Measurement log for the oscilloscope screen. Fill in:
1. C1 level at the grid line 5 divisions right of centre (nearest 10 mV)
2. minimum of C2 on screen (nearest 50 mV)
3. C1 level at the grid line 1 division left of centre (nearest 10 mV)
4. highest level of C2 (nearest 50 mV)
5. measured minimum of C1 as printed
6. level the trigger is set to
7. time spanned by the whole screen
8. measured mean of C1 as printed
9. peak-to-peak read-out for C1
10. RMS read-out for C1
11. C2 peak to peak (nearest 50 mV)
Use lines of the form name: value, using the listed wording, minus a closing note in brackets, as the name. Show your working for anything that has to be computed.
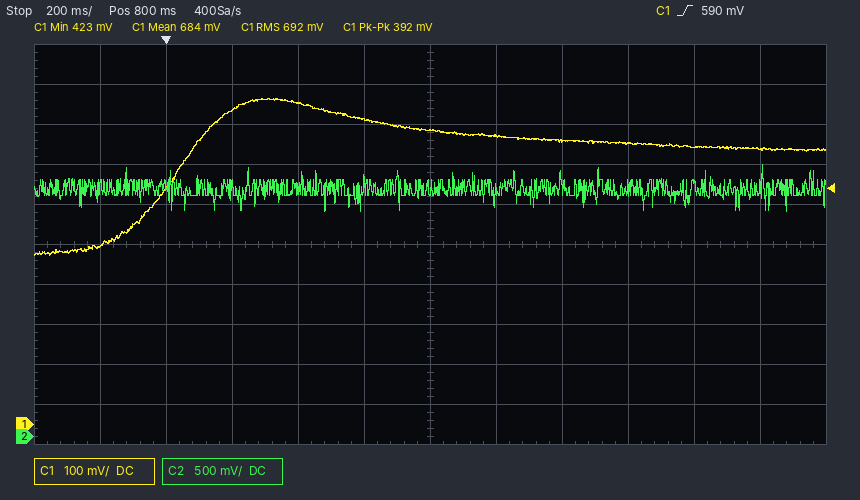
C1 level at the grid line 5 divisions right of centre: 690 mV
minimum of C2 on screen: 2.80 V
C1 level at the grid line 1 division left of centre: 760 mV
highest level of C2: 3.40 V
measured minimum of C1 as printed: 423 mV
level the trigger is set to: 590 mV
time spanned by the whole screen: 2.4 s
measured mean of C1 as printed: 684 mV
peak-to-peak read-out for C1: 392 mV
RMS read-out for C1: 692 mV
C2 peak to peak: 3.40 V − (2.80 V) = 600 mV
